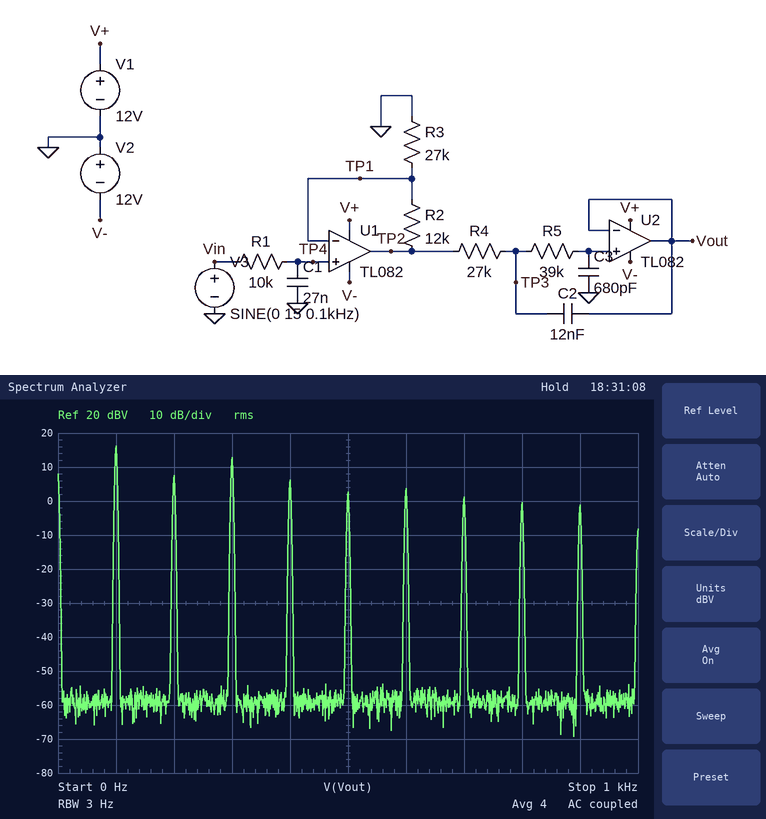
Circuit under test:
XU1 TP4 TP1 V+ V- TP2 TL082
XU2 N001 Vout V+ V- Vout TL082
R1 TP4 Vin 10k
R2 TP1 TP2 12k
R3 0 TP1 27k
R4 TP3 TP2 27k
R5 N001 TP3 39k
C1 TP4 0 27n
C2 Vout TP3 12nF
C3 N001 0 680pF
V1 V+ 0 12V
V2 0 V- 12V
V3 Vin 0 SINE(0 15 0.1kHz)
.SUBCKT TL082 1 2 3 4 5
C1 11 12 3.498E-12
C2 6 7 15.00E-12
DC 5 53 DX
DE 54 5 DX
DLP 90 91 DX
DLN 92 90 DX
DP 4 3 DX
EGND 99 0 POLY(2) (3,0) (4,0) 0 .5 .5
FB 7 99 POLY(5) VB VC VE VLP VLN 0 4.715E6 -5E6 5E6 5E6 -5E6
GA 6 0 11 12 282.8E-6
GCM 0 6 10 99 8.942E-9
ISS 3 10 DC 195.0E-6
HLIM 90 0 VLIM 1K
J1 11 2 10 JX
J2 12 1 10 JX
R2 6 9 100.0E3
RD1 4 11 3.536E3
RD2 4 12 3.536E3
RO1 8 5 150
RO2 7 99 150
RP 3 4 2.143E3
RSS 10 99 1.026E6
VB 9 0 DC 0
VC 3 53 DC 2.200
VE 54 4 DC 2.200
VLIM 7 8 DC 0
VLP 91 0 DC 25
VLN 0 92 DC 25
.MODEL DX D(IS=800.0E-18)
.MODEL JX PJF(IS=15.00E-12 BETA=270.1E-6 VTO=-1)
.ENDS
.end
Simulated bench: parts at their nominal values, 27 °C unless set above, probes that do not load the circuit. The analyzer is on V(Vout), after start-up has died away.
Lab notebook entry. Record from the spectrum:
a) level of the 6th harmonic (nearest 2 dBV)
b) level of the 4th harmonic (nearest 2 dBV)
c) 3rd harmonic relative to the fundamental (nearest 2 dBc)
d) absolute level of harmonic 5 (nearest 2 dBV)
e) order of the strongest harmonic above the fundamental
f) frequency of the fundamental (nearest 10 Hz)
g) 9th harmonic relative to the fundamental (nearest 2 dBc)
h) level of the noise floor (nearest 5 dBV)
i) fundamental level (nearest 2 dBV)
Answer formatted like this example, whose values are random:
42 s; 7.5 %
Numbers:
4 dBV; 6 dBV; -4 dBc; 2 dBV; 3; 100 Hz; -18 dBc; -60 dBV; 16 dBV
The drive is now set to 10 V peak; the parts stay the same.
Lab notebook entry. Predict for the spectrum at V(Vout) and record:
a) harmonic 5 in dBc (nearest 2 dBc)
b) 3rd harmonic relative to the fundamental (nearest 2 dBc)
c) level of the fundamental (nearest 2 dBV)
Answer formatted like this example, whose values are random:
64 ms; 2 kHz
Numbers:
-30 dBc; -18 dBc; 18 dBV
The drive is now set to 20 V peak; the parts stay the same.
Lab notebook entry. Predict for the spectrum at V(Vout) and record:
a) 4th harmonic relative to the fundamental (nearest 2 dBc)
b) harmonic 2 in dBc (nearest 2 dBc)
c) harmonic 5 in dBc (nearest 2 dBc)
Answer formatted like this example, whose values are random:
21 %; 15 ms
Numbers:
-18 dBc; 4 dBc; -2 dBc
